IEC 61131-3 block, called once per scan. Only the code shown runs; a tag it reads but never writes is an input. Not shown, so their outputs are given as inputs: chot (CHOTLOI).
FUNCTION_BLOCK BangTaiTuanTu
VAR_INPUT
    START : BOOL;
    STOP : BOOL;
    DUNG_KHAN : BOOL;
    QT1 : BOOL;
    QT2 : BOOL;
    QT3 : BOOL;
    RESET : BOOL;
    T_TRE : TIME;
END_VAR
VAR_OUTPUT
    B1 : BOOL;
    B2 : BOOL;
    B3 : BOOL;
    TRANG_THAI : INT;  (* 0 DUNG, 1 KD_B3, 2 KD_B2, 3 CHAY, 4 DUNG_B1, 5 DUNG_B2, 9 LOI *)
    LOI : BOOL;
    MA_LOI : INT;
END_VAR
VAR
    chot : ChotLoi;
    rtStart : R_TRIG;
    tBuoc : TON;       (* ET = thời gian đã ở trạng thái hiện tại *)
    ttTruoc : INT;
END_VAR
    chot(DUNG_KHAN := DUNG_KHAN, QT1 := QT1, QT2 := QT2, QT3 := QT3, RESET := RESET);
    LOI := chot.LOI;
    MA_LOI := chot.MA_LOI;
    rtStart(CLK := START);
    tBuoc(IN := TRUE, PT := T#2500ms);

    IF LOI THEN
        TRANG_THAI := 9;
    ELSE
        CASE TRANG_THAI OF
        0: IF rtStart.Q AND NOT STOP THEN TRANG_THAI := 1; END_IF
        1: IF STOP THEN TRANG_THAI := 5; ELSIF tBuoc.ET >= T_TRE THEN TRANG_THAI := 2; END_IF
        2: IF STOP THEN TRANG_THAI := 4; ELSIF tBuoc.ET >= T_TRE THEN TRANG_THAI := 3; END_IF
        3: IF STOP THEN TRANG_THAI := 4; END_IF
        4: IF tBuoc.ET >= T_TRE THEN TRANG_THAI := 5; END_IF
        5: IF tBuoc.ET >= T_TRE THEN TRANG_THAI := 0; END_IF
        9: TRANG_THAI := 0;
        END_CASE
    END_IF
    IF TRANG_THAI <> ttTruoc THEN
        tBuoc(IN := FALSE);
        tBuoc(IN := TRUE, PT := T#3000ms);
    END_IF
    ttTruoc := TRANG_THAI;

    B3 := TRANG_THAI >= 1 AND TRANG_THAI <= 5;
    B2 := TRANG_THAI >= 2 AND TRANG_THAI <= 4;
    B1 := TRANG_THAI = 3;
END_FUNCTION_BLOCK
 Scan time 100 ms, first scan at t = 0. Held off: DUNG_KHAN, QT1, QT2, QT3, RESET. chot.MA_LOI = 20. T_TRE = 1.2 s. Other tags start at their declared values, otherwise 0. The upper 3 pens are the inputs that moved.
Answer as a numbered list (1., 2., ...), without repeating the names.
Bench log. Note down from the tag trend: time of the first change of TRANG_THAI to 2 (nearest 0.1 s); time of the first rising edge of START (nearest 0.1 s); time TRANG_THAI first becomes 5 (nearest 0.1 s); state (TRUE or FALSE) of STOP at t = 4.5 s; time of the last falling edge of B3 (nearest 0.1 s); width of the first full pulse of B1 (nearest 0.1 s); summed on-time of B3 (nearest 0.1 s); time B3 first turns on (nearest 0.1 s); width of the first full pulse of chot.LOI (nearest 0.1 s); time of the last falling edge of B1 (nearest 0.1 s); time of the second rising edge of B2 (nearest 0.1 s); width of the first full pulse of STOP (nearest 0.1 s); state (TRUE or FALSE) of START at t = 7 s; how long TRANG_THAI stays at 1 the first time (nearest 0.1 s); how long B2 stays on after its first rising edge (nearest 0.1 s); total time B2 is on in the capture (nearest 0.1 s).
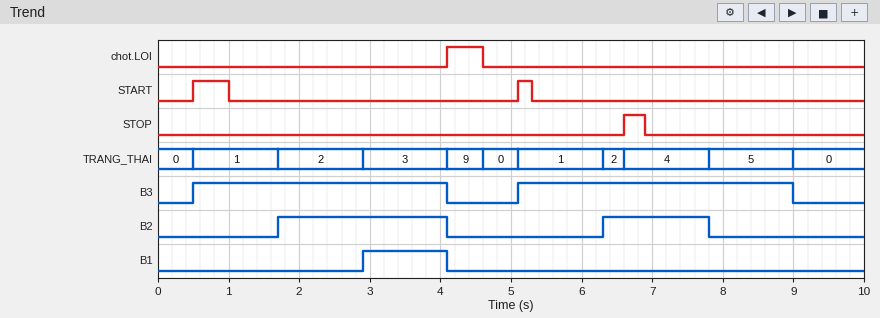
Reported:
1. 1.7 s
2. 0.5 s
3. 7.8 s
4. FALSE
5. 9.0 s
6. 1.2 s
7. 7.5 s
8. 0.5 s
9. 0.5 s
10. 4.1 s
11. 6.3 s
12. 0.3 s
13. FALSE
14. 1.2 s
15. 2.4 s
16. 3.9 s
